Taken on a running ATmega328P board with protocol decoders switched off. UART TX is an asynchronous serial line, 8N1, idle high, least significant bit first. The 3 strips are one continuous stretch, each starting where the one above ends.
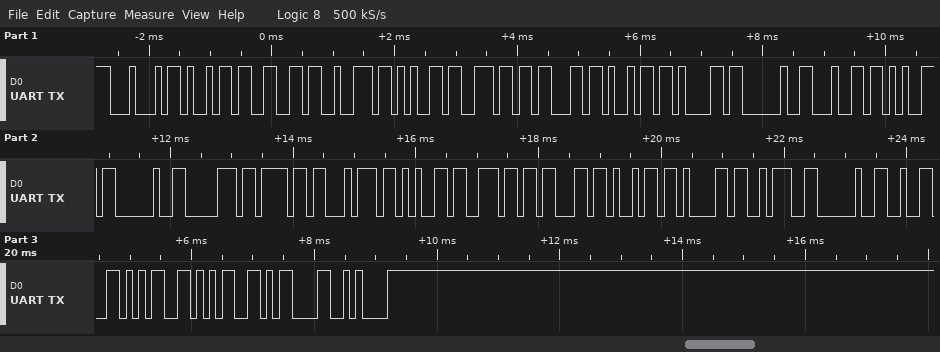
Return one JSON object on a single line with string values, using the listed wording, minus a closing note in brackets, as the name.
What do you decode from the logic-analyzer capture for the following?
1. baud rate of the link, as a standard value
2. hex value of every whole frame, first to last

{"baud rate of the link, as a standard value": "9600 baud", "hex value of every whole frame, first to last": "44 69 66 72 65 6E 63 69 61 20 64 65 20 70 6F 74 65 6E 63 69 61 3A 20 32 35 35 0D 0A"}
